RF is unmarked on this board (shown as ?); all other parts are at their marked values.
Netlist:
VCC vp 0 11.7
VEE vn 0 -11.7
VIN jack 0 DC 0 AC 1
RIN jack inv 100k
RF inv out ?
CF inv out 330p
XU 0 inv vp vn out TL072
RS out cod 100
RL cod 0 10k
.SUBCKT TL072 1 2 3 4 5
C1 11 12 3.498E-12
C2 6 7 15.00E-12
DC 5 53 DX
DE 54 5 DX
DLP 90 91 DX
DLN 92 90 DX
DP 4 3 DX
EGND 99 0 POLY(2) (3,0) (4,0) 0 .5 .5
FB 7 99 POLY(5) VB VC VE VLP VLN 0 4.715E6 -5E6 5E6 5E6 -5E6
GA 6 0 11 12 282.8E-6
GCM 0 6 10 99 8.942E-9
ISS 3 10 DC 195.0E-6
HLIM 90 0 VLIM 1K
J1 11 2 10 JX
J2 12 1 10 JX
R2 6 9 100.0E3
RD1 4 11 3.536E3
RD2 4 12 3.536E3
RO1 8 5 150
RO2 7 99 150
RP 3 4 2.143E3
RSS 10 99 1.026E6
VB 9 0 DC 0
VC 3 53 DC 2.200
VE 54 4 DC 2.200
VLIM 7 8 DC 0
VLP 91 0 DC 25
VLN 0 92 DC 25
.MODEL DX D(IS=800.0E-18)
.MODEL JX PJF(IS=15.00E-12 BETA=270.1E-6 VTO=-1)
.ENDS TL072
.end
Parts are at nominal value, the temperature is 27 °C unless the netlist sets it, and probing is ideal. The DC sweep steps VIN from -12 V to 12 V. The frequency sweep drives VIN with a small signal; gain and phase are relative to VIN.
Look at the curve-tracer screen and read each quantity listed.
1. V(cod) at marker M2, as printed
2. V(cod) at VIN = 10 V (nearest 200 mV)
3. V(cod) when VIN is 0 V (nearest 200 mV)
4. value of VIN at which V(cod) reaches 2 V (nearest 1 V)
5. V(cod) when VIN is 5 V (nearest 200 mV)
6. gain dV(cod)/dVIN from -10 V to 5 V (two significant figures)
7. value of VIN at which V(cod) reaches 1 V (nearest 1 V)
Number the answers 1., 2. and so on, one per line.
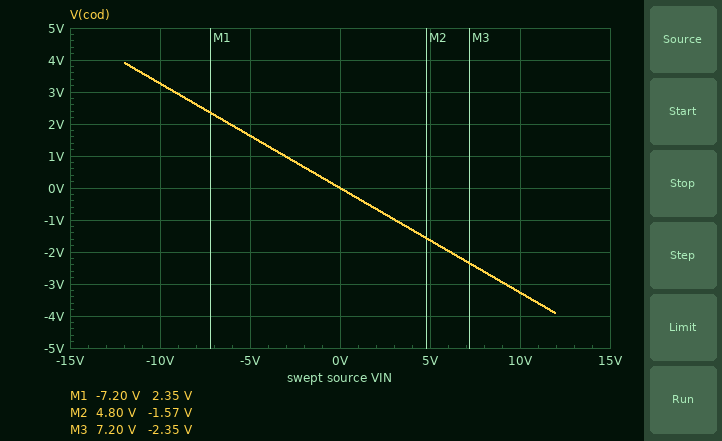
1. -1.57 V
2. -3.2 V
3. 0 V
4. -6 V
5. -1.6 V
6. -0.33 V/V
7. -3 V
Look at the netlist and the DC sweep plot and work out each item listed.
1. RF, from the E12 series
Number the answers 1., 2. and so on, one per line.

1. 33 kΩ
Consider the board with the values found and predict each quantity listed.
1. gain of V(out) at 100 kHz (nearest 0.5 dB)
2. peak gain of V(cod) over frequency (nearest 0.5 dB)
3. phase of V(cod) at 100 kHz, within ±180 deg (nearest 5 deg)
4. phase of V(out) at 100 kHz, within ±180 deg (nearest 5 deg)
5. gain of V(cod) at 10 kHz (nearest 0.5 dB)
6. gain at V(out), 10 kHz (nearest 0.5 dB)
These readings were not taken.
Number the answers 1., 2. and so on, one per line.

1. -26.5 dB
2. -9.5 dB
3. 95 deg
4. 95 deg
5. -11.5 dB
6. -11.5 dB
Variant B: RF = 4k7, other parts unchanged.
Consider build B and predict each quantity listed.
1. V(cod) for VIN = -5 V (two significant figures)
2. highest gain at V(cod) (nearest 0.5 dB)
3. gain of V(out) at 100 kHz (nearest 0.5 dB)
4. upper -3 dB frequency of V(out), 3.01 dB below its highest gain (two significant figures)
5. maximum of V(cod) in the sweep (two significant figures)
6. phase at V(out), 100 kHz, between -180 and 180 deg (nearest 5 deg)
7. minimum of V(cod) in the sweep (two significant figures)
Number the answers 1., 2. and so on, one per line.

1. 230 mV
2. -26.5 dB
3. -29.5 dB
4. 100 kHz
5. 560 mV
6. 135 deg
7. -560 mV
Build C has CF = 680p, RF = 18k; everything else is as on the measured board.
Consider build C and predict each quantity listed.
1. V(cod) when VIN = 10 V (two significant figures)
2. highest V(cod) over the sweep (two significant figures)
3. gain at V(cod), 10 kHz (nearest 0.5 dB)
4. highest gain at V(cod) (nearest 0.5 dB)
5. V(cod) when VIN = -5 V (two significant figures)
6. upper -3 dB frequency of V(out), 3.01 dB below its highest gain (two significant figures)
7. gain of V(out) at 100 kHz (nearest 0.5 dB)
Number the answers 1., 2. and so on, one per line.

1. -1.8 V
2. 2.1 V
3. -17.0 dB
4. -15.0 dB
5. 890 mV
6. 13 kHz
7. -32.5 dB
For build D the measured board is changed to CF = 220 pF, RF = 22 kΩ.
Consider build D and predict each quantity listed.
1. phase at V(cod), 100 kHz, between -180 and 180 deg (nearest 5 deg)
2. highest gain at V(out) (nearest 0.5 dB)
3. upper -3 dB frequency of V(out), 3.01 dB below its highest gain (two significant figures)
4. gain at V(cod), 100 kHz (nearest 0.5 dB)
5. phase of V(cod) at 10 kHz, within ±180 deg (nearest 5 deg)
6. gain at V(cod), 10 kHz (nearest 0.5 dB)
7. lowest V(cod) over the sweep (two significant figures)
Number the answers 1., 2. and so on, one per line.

1. 105 deg
2. -13.0 dB
3. 33 kHz
4. -23.5 dB
5. 165 deg
6. -13.5 dB
7. -2.6 V
